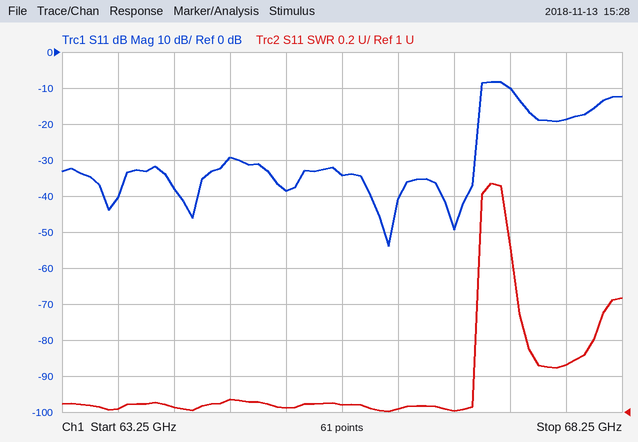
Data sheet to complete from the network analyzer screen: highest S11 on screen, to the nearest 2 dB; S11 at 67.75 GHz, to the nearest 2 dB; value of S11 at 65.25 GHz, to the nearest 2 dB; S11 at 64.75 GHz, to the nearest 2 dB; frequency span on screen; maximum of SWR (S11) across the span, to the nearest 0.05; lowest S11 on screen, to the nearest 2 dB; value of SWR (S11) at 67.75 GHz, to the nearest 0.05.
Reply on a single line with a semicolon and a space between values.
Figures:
-8 dB; -18 dB; -38 dB; -30 dB; 5 GHz; 2.25; -54 dB; 1.25
